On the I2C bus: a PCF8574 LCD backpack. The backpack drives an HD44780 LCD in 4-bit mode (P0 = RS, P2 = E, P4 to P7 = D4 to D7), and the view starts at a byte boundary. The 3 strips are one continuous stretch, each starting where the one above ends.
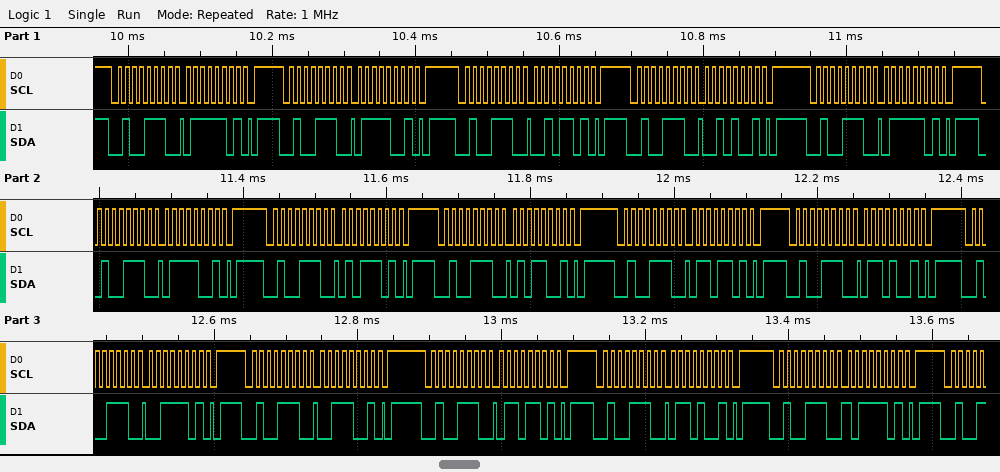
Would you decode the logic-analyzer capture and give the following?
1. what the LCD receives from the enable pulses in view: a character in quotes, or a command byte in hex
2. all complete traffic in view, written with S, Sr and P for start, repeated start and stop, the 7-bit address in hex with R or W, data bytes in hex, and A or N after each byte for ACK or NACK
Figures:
'r' 'u' 'c'
S 27W A 7D A P S 27W A 79 A P S 27W A 2D A P S 27W A 29 A P S 27W A 7D A P S 27W A 79 A P S 27W A 5D A P S 27W A 59 A P S 27W A 6D A P S 27W A 69 A P S 27W A 3D A P S 27W A 39 A P S 27W A 6D A P S 27W A 69 A P S 27W A BD A P
